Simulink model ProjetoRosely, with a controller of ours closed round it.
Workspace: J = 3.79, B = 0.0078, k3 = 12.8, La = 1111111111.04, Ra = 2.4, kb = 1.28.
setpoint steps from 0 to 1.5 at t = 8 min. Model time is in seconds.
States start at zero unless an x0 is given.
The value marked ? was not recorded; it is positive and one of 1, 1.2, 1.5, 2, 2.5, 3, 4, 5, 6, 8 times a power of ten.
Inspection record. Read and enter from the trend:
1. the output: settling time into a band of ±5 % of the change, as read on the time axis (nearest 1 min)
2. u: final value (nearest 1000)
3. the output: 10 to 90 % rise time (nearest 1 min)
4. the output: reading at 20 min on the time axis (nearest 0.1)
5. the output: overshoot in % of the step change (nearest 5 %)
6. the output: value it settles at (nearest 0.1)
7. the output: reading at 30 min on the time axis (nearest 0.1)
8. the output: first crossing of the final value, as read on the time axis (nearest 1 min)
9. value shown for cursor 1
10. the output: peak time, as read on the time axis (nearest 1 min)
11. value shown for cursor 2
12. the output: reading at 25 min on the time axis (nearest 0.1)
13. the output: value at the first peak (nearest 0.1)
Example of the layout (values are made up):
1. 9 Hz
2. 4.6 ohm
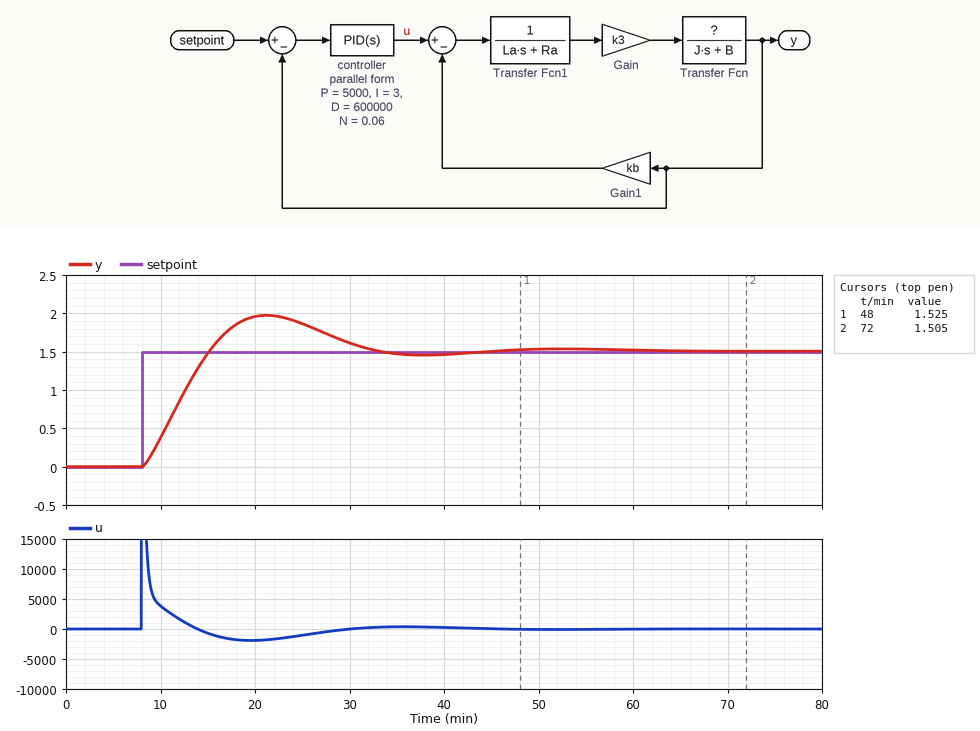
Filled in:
1. 31 min
2. 0
3. 5 min
4. 2.0
5. 30 %
6. 1.5
7. 1.6
8. 15 min
9. 1.525
10. 21 min
11. 1.505
12. 1.9
13. 2.0
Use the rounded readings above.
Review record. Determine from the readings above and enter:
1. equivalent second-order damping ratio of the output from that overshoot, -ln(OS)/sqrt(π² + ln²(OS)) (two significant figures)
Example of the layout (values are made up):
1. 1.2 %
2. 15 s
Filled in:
1. 0.36
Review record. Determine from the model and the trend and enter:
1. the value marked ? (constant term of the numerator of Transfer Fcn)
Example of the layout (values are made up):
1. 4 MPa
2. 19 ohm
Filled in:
1. 1
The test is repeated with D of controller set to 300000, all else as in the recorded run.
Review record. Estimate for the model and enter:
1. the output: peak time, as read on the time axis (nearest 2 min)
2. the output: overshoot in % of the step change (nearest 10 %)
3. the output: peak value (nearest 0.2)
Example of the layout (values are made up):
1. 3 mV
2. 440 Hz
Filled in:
1. 22 min
2. 40 %
3. 2.2
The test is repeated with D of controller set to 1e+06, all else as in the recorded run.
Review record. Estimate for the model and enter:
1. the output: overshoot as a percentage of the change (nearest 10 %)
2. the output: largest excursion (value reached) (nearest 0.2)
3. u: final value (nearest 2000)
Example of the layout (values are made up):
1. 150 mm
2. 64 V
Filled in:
1. 20 %
2. 1.8
3. 0
